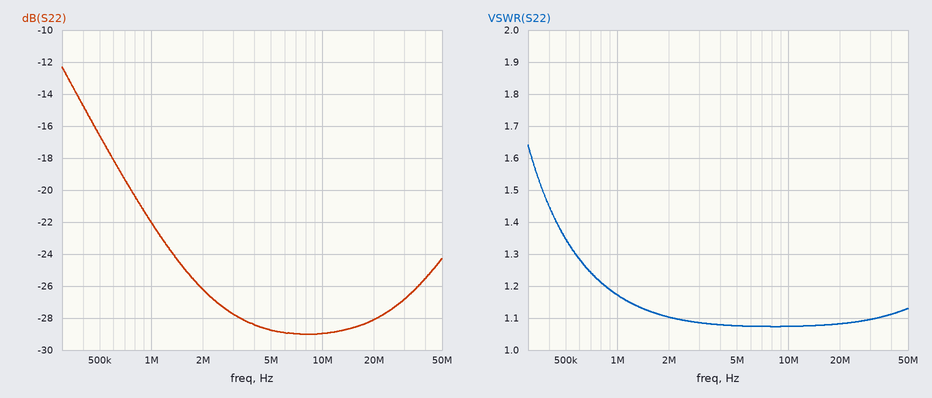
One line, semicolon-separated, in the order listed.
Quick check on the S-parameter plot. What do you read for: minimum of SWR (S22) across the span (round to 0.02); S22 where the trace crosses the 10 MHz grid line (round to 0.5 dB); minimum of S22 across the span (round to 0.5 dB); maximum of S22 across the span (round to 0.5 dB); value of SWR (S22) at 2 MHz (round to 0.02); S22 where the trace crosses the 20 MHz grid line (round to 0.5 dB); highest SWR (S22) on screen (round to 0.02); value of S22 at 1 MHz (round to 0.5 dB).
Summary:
1.08; -29.0 dB; -29.0 dB; -12.5 dB; 1.10; -28.0 dB; 1.64; -22.0 dB
